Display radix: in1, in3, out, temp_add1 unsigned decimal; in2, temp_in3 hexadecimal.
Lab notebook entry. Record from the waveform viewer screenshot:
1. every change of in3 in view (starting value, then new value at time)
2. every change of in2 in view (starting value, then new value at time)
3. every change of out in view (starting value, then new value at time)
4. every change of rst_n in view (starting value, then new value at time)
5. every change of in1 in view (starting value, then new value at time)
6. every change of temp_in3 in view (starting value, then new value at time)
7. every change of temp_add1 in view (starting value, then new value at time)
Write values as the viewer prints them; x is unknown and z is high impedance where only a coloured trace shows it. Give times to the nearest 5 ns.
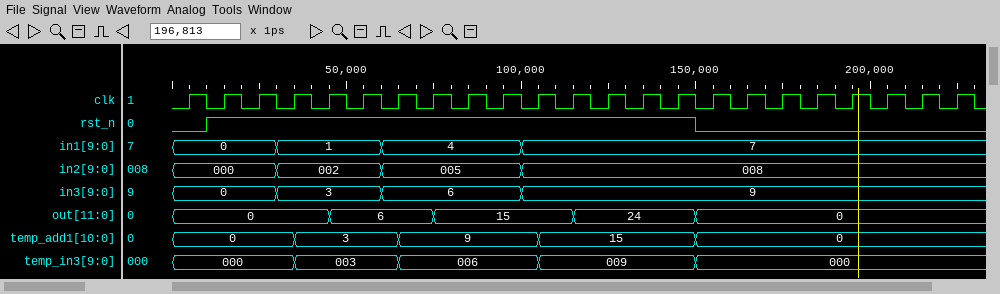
0, 3 at 30 ns, 6 at 60 ns, 9 at 100 ns
000, 002 at 30 ns, 005 at 60 ns, 008 at 100 ns
0, 6 at 45 ns, 15 at 75 ns, 24 at 115 ns, 0 at 150 ns
0, 1 at 10 ns, 0 at 150 ns
0, 1 at 30 ns, 4 at 60 ns, 7 at 100 ns
000, 003 at 35 ns, 006 at 65 ns, 009 at 105 ns, 000 at 150 ns
0, 3 at 35 ns, 9 at 65 ns, 15 at 105 ns, 0 at 150 ns
